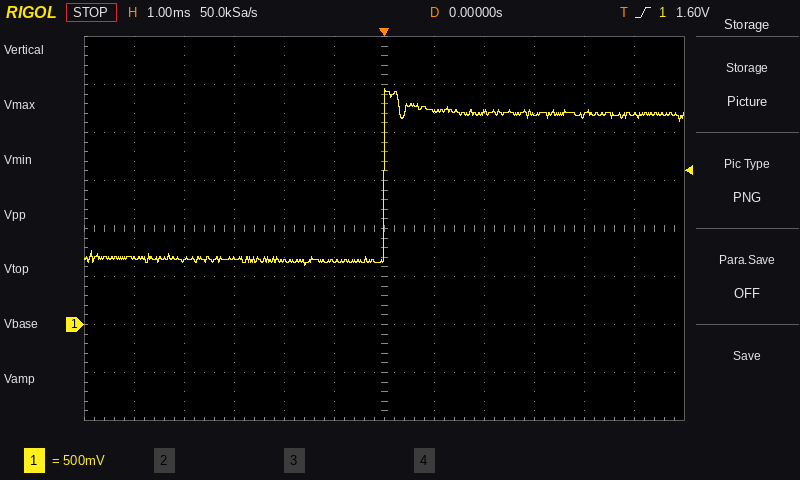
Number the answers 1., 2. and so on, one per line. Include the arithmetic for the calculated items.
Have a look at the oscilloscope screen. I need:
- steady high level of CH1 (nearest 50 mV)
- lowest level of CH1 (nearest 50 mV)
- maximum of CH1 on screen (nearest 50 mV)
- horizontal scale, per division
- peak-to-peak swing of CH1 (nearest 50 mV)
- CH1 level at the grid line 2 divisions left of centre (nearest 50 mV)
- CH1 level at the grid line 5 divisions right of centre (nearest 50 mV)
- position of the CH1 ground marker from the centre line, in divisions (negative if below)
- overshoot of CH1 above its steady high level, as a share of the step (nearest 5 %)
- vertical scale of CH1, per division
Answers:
1. 2.20 V
2. 600 mV
3. 2.45 V
4. 1 ms
5. 2.45 V − (600 mV) = 1.85 V
6. 650 mV
7. 2.20 V
8. -2.0 div
9. 15 %
10. 500 mV
